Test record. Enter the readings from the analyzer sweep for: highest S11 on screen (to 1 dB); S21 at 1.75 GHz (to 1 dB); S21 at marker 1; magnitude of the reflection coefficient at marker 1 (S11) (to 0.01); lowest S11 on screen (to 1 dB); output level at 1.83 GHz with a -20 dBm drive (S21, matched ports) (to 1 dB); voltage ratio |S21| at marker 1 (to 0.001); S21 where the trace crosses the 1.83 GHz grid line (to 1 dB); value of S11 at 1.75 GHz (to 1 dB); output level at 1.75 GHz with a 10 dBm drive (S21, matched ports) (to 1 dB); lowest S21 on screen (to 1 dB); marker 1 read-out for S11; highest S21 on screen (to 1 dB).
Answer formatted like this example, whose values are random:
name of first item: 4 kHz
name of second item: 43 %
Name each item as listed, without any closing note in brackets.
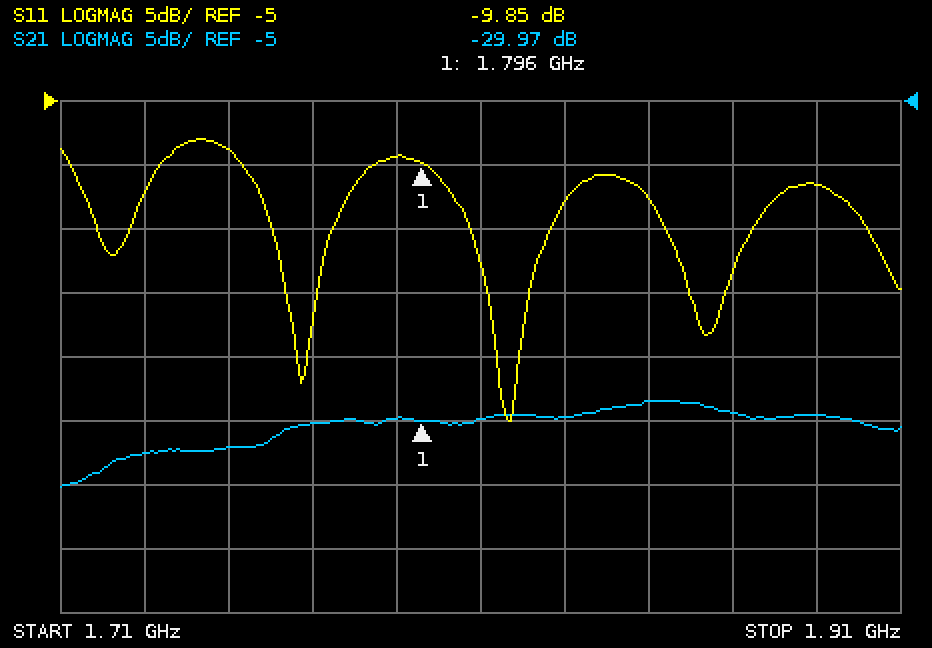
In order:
highest S11 on screen: -8 dB
S21 at 1.75 GHz: -32 dB
S21 at marker 1: -29.97 dB
magnitude of the reflection coefficient at marker 1 (S11): 0.32
lowest S11 on screen: -30 dB
output level at 1.83 GHz with a -20 dBm drive (S21, matched ports): -50 dBm
voltage ratio |S21| at marker 1: 0.032
S21 where the trace crosses the 1.83 GHz grid line: -30 dB
value of S11 at 1.75 GHz: -9 dB
output level at 1.75 GHz with a 10 dBm drive (S21, matched ports): -22 dBm
lowest S21 on screen: -35 dB
marker 1 read-out for S11: -9.85 dB
highest S21 on screen: -28 dB
